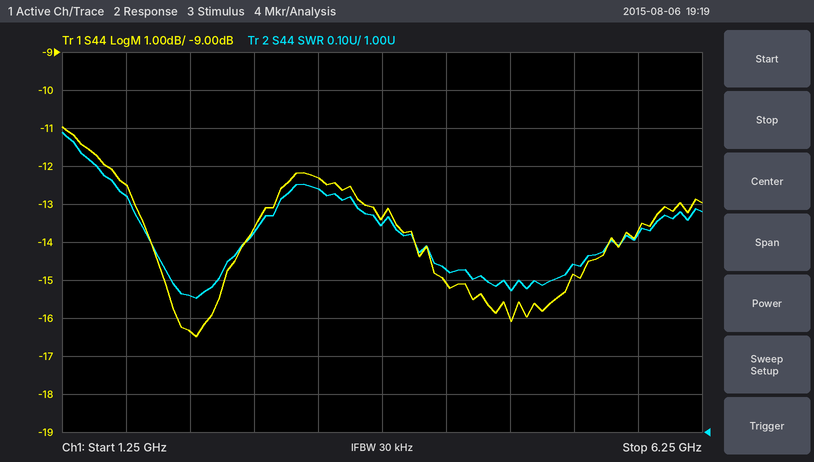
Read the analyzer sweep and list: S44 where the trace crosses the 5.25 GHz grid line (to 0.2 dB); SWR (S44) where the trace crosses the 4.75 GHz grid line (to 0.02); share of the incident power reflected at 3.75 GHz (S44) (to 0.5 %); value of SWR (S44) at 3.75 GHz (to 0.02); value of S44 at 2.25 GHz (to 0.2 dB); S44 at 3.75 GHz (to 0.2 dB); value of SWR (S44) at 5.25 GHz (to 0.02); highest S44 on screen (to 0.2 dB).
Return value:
-14.8 dB
1.38
4.5 %
1.54
-16.4 dB
-13.4 dB
1.44
-11.0 dB
